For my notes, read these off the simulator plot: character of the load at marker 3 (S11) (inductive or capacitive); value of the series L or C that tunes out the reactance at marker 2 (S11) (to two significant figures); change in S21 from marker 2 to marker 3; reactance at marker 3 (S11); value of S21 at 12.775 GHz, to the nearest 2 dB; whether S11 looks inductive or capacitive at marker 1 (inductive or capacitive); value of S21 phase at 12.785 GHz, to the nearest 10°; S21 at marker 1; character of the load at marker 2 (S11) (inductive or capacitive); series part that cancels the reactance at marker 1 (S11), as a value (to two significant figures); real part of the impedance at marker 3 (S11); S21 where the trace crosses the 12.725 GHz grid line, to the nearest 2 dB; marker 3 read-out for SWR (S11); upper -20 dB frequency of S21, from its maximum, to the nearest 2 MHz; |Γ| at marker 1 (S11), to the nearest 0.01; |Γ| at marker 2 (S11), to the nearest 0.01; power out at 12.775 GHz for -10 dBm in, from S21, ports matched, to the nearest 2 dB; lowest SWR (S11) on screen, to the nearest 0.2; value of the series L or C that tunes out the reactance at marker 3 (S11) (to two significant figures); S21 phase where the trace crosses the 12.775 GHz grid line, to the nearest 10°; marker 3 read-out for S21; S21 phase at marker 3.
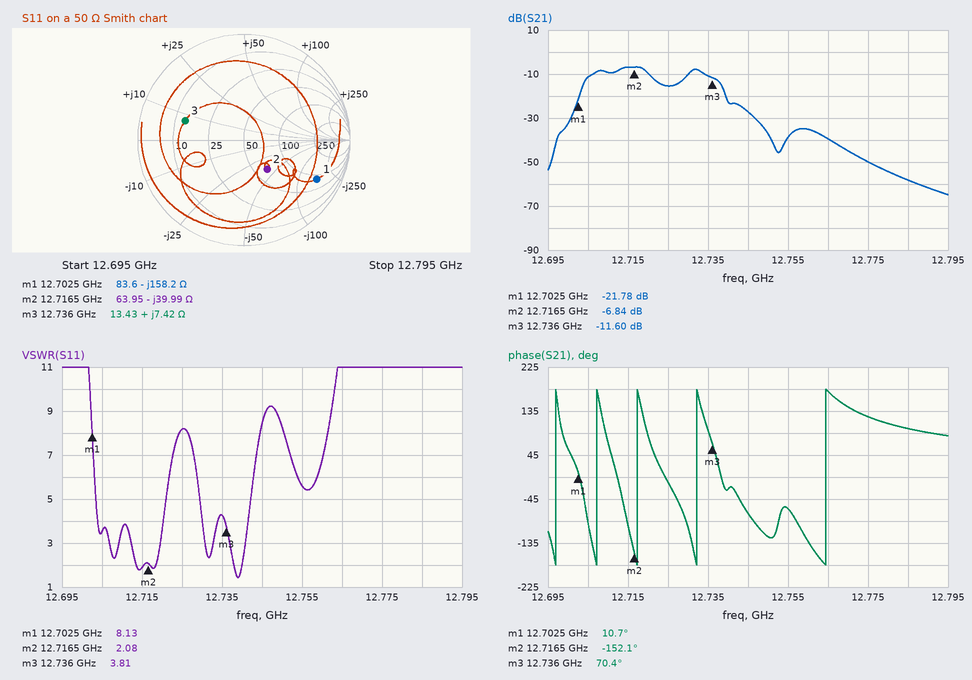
inductive
500 pH
-4.76 dB
+7.42 Ω
-50 dB
capacitive
100°
-21.78 dB
capacitive
2.0 nH
13.43 Ω
-16 dB
3.81
12.744 GHz
0.78
0.35
-60 dBm
1.4
1.7 pF
120°
-11.60 dB
70.4°
